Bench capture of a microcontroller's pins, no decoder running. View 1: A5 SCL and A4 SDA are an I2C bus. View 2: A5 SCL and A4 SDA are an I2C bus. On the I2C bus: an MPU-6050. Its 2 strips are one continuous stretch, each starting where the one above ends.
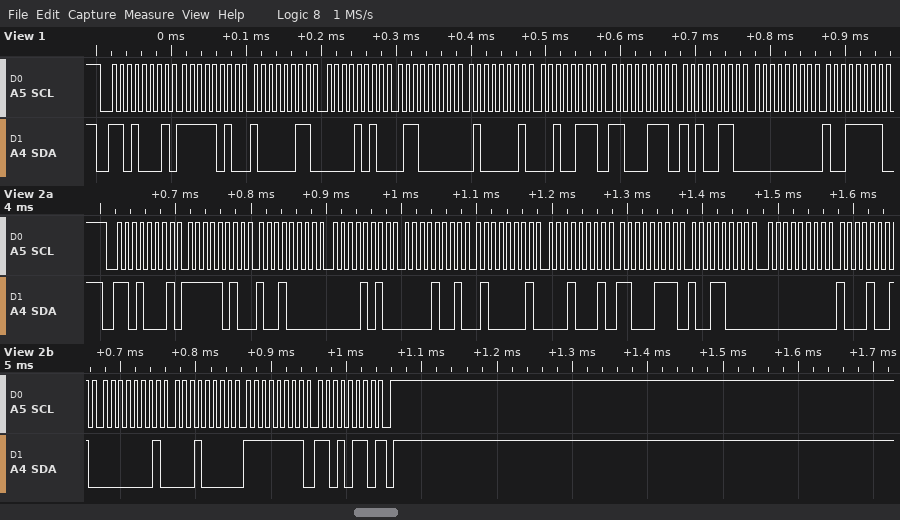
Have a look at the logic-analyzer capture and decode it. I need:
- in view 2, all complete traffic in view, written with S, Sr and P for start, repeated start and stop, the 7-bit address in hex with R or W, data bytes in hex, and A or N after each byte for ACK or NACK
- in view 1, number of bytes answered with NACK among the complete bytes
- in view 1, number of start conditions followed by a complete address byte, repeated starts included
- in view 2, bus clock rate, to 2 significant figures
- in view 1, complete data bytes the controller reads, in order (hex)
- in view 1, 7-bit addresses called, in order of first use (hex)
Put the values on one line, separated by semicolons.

S 68R A FA A 90 A 0A A 09 A 41 A 11 A C7 A 98 A 00 A 89 A 01 A 10 A FF A D6 N P; 0; 1; 100 kHz; FA 83 0A 60 41 27 C7 A6 00 9F; 0x68
